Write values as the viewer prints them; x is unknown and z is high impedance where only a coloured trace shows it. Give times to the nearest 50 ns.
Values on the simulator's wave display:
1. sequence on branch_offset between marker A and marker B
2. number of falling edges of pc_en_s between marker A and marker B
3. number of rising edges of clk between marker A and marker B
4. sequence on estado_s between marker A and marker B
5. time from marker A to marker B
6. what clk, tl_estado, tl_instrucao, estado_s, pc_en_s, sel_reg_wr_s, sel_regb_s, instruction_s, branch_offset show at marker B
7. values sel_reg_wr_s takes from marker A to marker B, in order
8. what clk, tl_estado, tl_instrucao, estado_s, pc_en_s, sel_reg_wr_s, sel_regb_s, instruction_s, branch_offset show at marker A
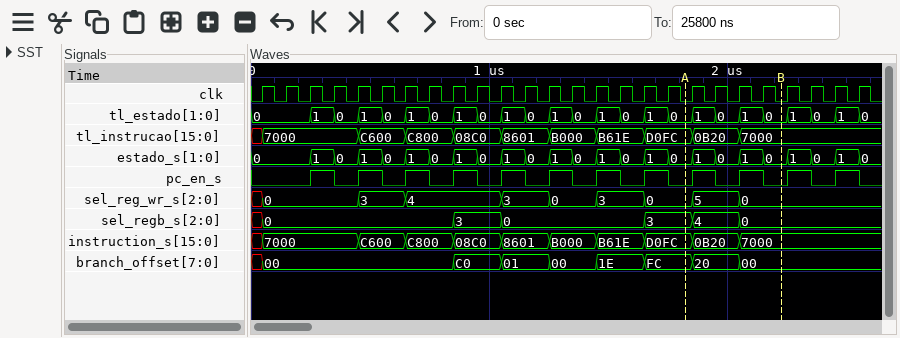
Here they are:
FC, 20, 00
2
4
0, 1, 0, 1, 0
400 ns
clk=0, tl_estado=0, tl_instrucao=7000, estado_s=0, pc_en_s=0, sel_reg_wr_s=0, sel_regb_s=0, instruction_s=7000, branch_offset=00
0, 5, 0
clk=0, tl_estado=0, tl_instrucao=D0FC, estado_s=0, pc_en_s=0, sel_reg_wr_s=0, sel_regb_s=3, instruction_s=D0FC, branch_offset=FC
